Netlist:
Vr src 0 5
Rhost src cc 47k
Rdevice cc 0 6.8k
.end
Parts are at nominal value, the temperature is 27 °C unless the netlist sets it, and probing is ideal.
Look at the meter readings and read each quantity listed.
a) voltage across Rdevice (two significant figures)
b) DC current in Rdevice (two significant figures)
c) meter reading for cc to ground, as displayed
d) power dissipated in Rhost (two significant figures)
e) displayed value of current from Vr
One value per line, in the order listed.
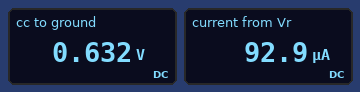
630 mV
93 µA
0.632 V
410 µW
92.9 µA
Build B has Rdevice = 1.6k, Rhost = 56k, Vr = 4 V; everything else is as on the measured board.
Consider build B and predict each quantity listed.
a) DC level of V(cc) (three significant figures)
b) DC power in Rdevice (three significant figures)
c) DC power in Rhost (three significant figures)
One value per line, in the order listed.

111 mV
7.72 µW
270 µW
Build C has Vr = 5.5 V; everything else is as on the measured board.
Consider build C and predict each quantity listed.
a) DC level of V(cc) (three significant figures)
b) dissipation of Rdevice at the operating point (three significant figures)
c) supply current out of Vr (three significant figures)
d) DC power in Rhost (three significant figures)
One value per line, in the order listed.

695 mV
71.1 µW
102 µA
491 µW
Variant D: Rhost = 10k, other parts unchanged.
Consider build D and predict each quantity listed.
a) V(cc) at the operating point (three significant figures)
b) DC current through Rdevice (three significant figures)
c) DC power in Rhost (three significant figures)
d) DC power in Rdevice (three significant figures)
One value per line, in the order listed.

2.02 V
298 µA
886 µW
602 µW
